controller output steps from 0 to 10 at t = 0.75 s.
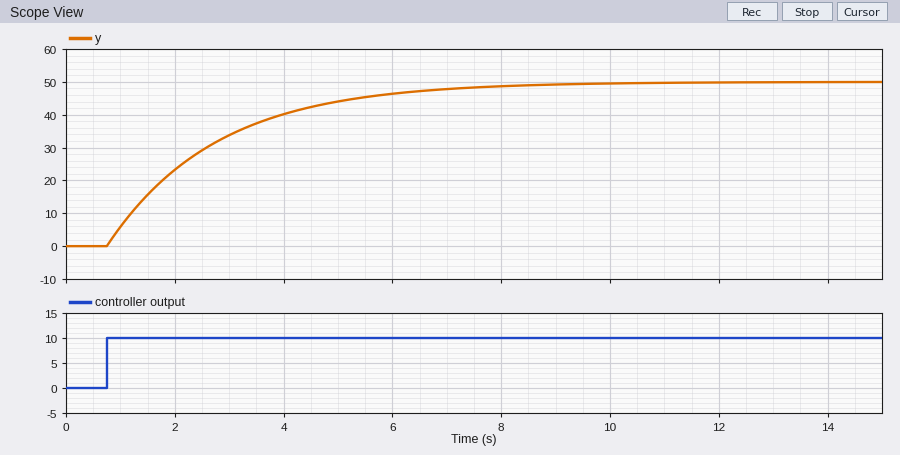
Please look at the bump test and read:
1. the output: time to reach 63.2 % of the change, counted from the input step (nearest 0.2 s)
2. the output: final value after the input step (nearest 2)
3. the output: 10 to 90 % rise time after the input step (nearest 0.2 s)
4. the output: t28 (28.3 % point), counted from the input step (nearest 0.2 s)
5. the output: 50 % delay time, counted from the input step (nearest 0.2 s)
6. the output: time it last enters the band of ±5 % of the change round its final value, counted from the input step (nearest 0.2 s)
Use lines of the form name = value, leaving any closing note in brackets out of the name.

the output: time to reach 63.2 % of the change, counted from the input step = 2.0 s
the output: final value after the input step = 50
the output: 10 to 90 % rise time after the input step = 4.4 s
the output: t28 (28.3 % point), counted from the input step = 0.6 s
the output: 50 % delay time, counted from the input step = 1.4 s
the output: time it last enters the band of ±5 % of the change round its final value, counted from the input step = 6.0 s
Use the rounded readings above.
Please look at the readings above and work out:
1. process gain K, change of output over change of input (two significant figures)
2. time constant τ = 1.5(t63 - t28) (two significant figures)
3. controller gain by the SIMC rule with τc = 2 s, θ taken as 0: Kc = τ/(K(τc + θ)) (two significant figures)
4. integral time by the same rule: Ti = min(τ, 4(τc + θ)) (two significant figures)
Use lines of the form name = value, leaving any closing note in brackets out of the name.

process gain K, change of output over change of input = 5.0
time constant τ = 1.5(t63 - t28) = 2.1 s
controller gain by the SIMC rule with τc = 2 s, θ taken as 0: Kc = τ/(K(τc + θ)) = 0.21
integral time by the same rule: Ti = min(τ, 4(τc + θ)) = 2.1 s
